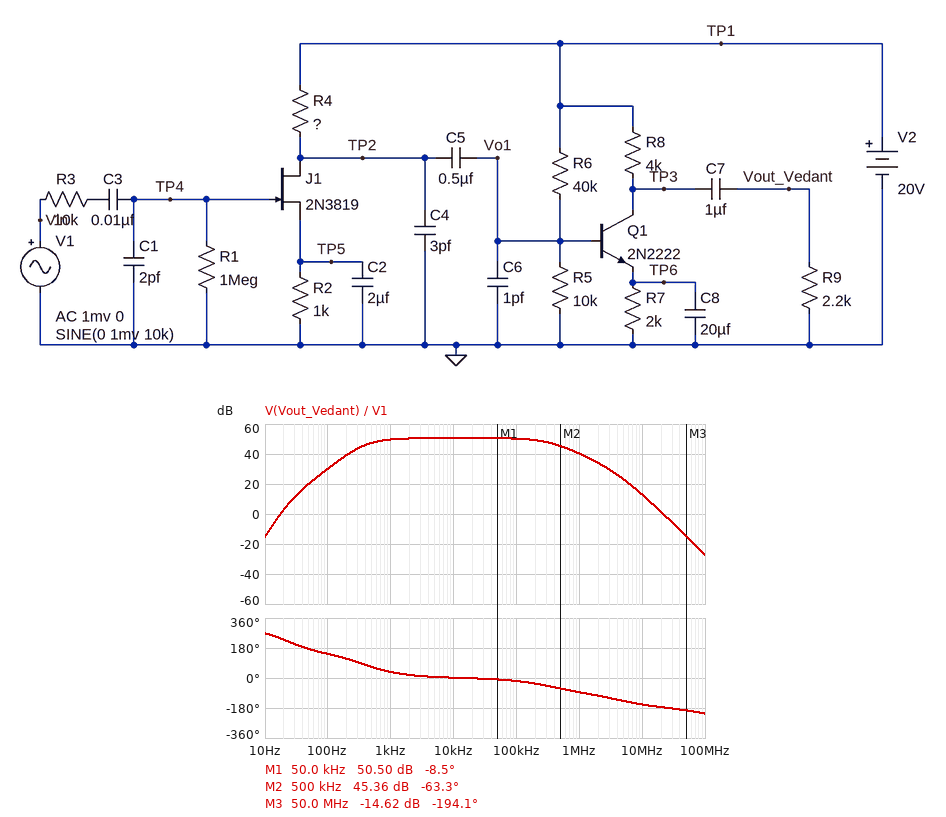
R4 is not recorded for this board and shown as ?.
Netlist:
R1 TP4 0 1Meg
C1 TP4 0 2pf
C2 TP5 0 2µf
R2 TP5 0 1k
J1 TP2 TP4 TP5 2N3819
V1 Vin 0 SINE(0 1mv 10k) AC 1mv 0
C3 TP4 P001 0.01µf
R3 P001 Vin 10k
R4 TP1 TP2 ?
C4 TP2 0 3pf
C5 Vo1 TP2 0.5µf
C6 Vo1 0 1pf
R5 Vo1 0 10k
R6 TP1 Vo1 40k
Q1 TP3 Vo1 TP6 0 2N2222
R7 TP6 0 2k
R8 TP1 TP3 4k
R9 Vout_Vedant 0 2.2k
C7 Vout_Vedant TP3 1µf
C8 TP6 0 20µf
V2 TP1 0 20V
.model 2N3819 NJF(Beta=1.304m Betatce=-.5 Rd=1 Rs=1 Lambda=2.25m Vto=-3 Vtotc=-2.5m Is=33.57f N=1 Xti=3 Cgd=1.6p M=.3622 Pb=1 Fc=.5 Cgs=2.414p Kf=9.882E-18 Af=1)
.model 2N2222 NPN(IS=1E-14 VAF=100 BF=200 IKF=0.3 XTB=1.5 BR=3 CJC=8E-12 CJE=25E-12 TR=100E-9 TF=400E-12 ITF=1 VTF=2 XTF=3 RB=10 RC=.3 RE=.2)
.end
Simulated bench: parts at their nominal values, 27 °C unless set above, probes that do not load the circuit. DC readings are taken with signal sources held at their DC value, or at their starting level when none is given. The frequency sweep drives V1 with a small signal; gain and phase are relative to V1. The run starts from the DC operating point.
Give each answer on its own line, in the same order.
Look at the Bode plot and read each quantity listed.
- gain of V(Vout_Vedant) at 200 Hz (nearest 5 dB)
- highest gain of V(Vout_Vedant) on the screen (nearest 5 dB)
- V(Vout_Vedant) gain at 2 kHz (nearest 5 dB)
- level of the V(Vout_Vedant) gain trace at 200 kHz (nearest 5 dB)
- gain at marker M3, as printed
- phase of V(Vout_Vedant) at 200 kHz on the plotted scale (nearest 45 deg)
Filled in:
40 dB
50 dB
50 dB
50 dB
-14.62 dB
-45 deg
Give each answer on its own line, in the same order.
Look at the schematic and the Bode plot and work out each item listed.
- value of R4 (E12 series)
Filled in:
2.7 kΩ
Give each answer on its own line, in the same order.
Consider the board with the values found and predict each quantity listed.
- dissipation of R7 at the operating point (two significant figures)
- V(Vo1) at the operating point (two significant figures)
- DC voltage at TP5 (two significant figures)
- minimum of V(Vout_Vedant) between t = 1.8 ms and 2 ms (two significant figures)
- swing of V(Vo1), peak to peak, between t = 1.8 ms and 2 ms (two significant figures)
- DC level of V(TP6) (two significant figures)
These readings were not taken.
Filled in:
5.4 mW
3.9 V
1.8 V
-340 mV
7.9 mV
3.3 V
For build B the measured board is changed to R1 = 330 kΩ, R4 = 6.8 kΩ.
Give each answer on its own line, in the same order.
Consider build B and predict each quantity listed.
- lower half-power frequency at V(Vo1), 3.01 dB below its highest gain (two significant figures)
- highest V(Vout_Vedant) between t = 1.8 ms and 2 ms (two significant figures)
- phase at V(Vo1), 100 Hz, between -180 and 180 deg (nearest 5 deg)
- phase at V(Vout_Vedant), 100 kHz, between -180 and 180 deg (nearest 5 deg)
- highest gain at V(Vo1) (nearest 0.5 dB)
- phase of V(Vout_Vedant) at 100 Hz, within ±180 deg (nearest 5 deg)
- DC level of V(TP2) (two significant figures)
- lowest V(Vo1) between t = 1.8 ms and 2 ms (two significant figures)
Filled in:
140 Hz
450 mV
-120 deg
-25 deg
15.0 dB
150 deg
7.6 V
3.9 V
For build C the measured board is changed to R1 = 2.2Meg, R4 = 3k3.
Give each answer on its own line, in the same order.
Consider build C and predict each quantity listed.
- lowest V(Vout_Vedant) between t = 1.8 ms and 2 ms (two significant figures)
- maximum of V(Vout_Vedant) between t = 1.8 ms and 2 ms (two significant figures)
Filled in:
-380 mV
360 mV
